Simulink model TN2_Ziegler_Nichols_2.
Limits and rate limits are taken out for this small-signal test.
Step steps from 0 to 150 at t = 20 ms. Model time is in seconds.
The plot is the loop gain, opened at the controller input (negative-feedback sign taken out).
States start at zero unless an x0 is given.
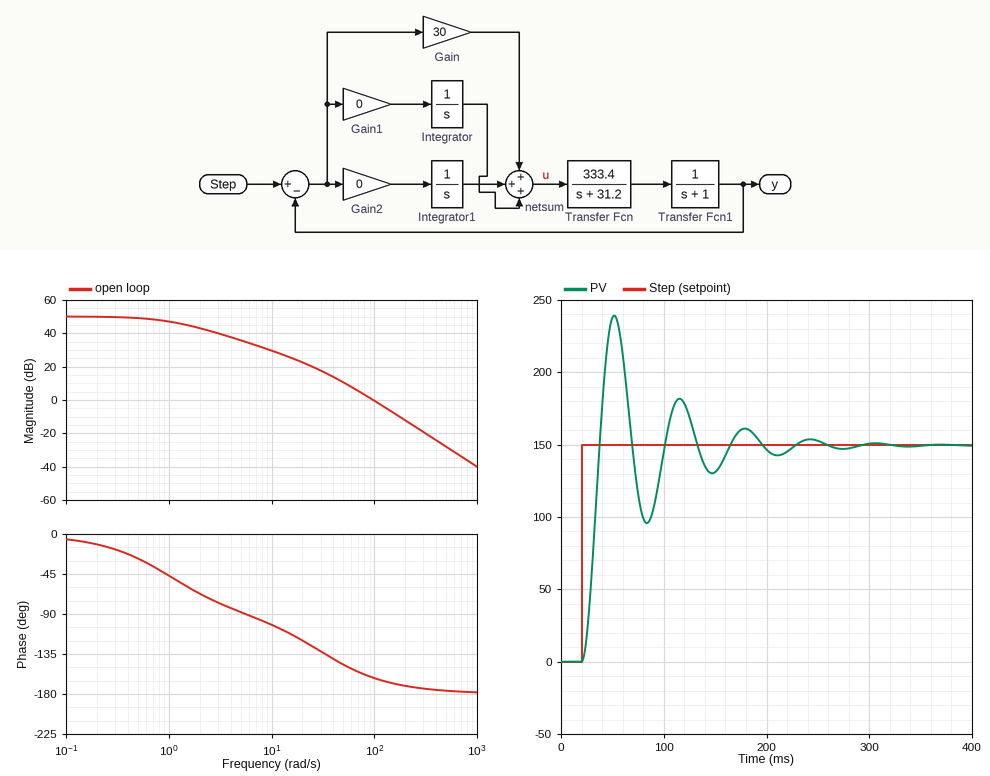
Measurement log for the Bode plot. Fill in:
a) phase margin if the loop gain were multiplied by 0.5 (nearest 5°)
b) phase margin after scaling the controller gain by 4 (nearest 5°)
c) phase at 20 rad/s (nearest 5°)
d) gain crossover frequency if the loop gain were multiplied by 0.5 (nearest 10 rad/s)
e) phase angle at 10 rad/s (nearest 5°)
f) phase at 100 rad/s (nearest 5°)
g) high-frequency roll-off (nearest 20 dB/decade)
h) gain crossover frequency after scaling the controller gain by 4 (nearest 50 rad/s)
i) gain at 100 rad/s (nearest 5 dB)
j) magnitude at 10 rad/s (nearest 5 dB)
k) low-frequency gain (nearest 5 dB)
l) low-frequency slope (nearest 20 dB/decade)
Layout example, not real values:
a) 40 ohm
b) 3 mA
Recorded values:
a) 25°
b) 10°
c) -120°
d) 70 rad/s
e) -100°
f) -160°
g) -40 dB/decade
h) 200 rad/s
i) 0 dB
j) 30 dB
k) 50 dB
l) 0 dB/decade
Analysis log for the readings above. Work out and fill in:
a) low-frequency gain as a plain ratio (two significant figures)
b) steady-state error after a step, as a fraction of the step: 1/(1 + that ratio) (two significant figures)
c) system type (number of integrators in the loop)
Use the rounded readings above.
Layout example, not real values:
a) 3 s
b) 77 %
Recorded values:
a) 320
b) 0.0031
c) 0
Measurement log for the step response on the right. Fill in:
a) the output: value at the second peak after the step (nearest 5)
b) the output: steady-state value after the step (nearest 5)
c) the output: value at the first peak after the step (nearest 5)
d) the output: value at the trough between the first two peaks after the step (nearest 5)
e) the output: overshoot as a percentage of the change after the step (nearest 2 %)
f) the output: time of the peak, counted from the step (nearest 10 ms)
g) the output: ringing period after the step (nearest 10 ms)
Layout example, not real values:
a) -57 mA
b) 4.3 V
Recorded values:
a) 180
b) 150
c) 240
d) 95
e) 60 %
f) 30 ms
g) 60 ms
